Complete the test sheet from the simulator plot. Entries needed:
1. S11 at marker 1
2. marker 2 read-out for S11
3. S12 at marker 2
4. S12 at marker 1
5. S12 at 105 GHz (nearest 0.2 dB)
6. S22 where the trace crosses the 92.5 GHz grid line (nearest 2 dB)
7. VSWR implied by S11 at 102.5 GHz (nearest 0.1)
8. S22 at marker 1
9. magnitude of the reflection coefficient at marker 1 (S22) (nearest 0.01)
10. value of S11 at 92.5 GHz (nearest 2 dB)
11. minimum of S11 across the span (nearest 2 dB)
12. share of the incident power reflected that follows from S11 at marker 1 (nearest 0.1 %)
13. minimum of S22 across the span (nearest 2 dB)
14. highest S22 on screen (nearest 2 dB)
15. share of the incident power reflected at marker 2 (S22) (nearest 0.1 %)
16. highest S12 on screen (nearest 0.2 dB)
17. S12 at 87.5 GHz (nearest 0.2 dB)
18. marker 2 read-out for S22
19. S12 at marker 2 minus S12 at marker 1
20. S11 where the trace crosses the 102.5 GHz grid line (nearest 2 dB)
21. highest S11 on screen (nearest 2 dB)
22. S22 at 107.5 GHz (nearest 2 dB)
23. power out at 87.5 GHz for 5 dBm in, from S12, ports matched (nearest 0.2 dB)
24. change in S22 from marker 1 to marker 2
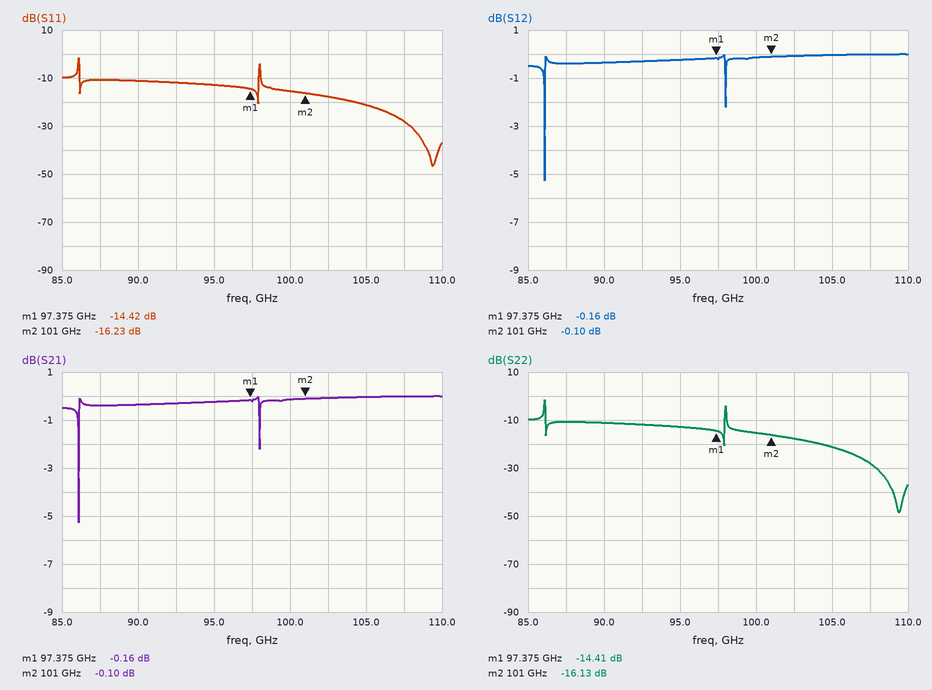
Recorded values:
-14.42 dB
-16.23 dB
-0.10 dB
-0.16 dB
0.0 dB
-12 dB
1.3
-14.41 dB
0.19
-12 dB
-46 dB
3.6 %
-48 dB
-2 dB
2.4 %
0.0 dB
-0.4 dB
-16.13 dB
0.06 dB
-18 dB
-2 dB
-28 dB
4.6 dBm
-1.72 dB
